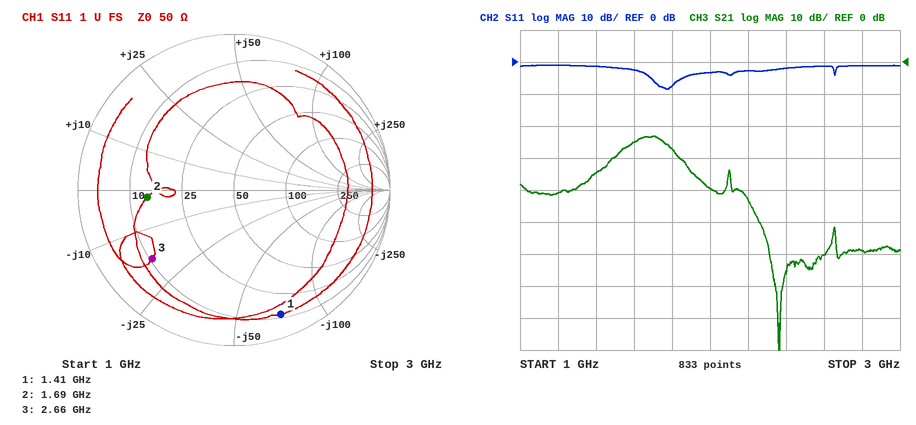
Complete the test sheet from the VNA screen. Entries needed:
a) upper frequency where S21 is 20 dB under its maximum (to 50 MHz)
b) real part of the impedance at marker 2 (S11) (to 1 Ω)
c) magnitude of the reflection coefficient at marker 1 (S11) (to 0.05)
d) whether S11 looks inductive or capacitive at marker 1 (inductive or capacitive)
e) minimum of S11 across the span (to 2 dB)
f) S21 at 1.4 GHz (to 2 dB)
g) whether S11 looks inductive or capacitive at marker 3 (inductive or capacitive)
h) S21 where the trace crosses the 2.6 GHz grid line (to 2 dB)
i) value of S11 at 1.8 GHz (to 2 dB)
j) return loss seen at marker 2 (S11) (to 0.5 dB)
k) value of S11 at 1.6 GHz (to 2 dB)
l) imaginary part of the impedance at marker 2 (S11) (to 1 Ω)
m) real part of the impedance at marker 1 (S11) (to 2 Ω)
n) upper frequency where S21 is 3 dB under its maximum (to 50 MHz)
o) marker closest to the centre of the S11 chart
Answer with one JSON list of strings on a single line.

["2.20 GHz", "14 Ω", "0.85", "capacitive", "-8 dB", "-34 dB", "capacitive", "-60 dB", "-8 dB", "5.0 dB", "-2 dB", "-2 Ω", "12 Ω", "1.80 GHz", "marker 2"]
